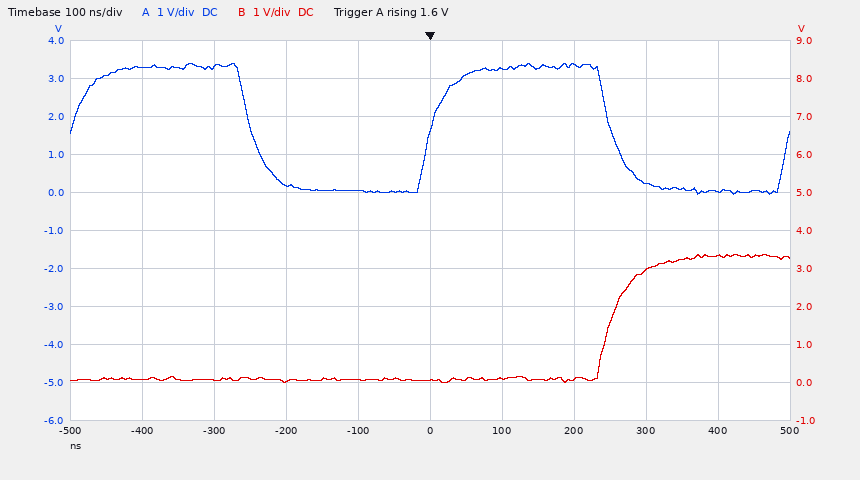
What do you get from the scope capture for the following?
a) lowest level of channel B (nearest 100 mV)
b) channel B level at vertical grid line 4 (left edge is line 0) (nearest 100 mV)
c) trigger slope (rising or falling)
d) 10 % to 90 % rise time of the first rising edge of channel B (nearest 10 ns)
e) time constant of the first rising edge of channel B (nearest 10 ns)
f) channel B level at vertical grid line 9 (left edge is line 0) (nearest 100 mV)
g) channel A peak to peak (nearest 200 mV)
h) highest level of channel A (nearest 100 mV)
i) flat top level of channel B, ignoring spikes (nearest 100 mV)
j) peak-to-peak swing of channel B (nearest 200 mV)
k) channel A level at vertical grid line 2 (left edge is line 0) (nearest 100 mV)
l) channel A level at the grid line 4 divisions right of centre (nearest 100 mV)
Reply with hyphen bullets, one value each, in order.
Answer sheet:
- 0.0 V
- 100 mV
- rising
- 70 ns
- 30 ns
- 3.3 V
- 3.4 V
- 3.4 V
- 3.3 V
- 3.4 V
- 3.3 V
- 0.0 V
